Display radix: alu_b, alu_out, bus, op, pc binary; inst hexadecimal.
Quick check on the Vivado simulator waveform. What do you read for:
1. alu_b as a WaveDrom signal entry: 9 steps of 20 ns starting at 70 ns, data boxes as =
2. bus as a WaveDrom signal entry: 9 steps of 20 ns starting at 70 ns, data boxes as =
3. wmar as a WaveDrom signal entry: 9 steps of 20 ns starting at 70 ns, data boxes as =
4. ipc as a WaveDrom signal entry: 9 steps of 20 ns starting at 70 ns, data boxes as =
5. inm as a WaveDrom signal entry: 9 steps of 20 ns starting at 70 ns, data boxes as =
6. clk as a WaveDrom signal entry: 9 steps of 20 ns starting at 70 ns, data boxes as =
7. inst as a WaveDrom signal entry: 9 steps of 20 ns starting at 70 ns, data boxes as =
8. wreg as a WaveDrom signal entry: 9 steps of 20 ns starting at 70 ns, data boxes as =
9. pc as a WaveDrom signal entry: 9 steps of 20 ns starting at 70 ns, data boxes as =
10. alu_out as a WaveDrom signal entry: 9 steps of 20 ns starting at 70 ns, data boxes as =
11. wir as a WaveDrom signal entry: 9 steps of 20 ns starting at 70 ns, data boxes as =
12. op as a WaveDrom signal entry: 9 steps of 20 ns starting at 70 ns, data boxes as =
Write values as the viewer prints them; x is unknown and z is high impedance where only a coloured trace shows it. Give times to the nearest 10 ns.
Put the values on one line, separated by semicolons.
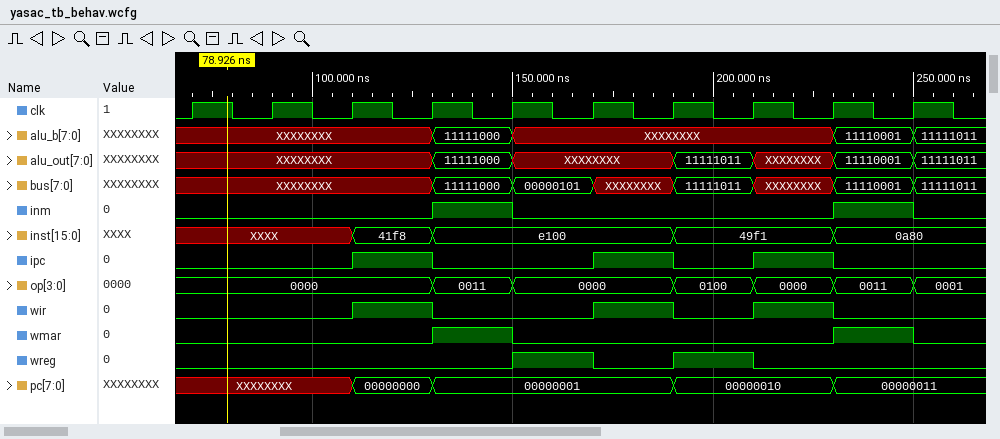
{name: 'alu_b', wave: 'x..=x...=', data: '11111000 11110001'}; {name: 'bus', wave: 'x..==x=x=', data: '11111000 00000101 11111011 11110001'}; {name: 'wmar', wave: '0..10...1'}; {name: 'ipc', wave: '0.10.1010'}; {name: 'inm', wave: '0..10...1'}; {name: 'clk', wave: 'p........'}; {name: 'inst', wave: 'x.==..=.=', data: '41f8 e100 49f1 0a80'}; {name: 'wreg', wave: '0...1010.'}; {name: 'pc', wave: 'x.==..=.=', data: '00000000 00000001 00000010 00000011'}; {name: 'alu_out', wave: 'x..=x.=x=', data: '11111000 11111011 11110001'}; {name: 'wir', wave: '0.10.1010'}; {name: 'op', wave: '=..==.===', data: '0000 0011 0000 0100 0000 0011'}
